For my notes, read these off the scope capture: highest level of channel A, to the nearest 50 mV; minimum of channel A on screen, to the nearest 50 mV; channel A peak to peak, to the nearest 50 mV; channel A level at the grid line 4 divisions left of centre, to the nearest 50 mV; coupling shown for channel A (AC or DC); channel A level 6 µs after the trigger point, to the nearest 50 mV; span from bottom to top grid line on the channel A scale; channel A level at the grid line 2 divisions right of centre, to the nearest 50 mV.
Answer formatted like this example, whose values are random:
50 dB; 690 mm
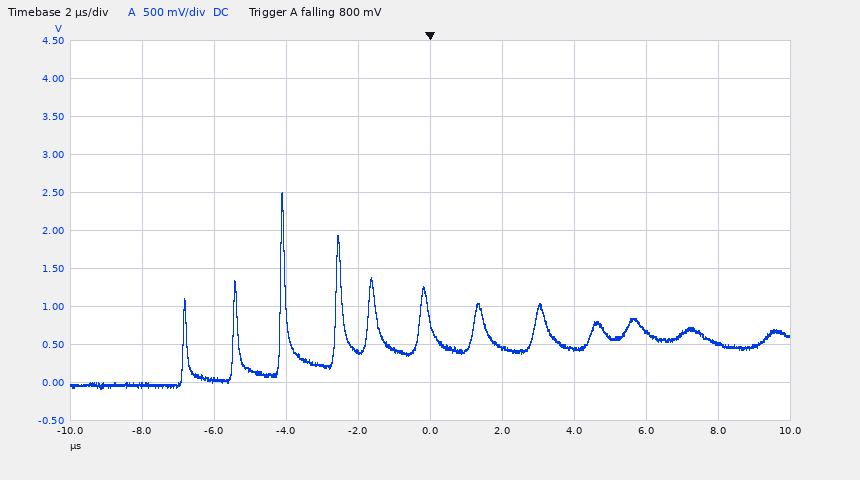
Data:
2.50 V; -100 mV; 2.60 V; -50 mV; DC; 700 mV; 5 V; 450 mV
